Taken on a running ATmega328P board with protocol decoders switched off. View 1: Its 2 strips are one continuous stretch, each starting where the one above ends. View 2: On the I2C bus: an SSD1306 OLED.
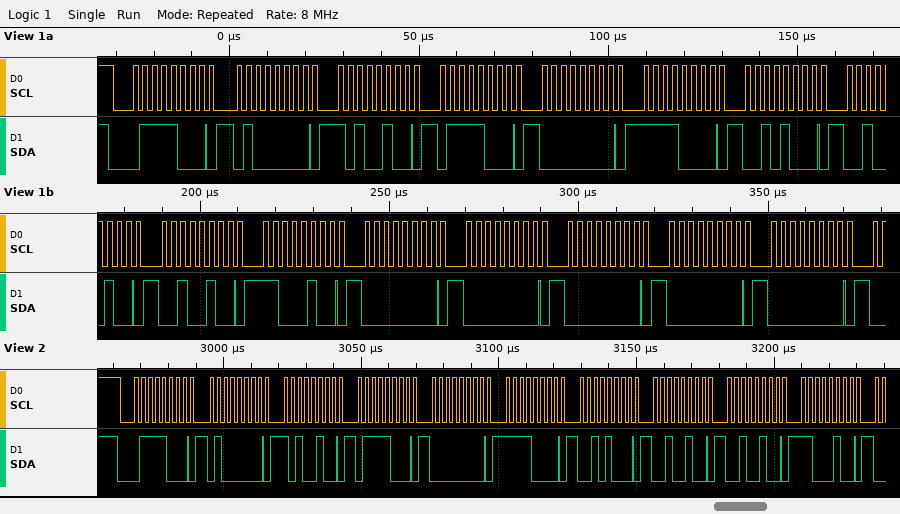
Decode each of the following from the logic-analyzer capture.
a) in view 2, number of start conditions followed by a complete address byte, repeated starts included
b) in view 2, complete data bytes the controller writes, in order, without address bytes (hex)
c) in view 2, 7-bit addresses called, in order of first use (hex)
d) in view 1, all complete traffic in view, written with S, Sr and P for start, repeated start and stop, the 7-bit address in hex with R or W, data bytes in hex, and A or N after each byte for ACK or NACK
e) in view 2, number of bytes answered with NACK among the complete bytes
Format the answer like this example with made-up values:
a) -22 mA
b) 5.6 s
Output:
a) 1
b) 40 A4 78 00 F0 28 24 24 C4
c) 0x3C
d) S 3CW A 40 A A4 A 78 A 00 A F0 A 28 A 24 A 24 A C4 A 00 A 00 A 00 A 00 A 00 A
e) 0
